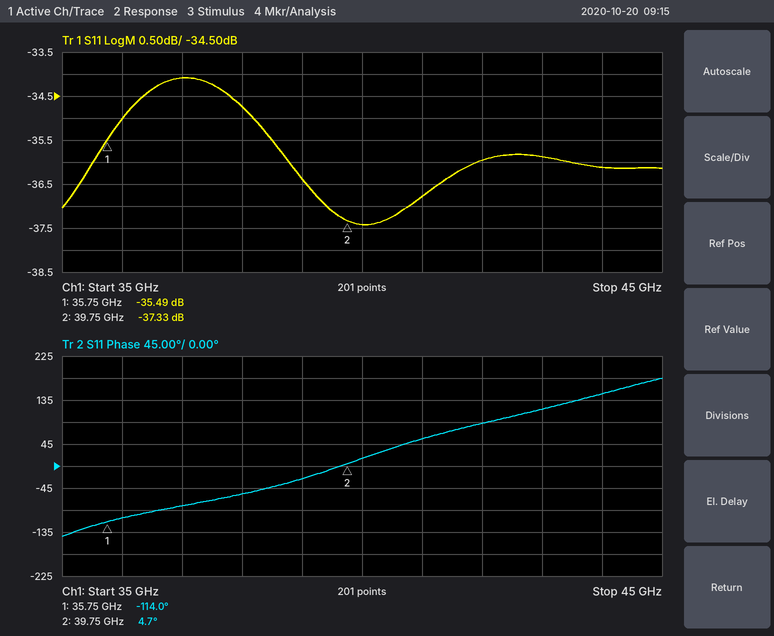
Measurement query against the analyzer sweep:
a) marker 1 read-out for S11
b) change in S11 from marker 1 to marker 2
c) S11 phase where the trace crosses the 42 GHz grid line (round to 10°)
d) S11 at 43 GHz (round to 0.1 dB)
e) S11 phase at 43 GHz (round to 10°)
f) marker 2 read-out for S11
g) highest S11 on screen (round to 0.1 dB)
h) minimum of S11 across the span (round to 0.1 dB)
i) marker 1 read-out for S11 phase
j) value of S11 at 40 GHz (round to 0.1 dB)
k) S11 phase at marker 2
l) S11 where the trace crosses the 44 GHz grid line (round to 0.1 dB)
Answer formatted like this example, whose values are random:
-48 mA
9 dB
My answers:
-35.49 dB
-1.84 dB
90°
-35.9 dB
120°
-37.33 dB
-34.1 dB
-37.4 dB
-114.0°
-37.4 dB
4.7°
-36.1 dB
